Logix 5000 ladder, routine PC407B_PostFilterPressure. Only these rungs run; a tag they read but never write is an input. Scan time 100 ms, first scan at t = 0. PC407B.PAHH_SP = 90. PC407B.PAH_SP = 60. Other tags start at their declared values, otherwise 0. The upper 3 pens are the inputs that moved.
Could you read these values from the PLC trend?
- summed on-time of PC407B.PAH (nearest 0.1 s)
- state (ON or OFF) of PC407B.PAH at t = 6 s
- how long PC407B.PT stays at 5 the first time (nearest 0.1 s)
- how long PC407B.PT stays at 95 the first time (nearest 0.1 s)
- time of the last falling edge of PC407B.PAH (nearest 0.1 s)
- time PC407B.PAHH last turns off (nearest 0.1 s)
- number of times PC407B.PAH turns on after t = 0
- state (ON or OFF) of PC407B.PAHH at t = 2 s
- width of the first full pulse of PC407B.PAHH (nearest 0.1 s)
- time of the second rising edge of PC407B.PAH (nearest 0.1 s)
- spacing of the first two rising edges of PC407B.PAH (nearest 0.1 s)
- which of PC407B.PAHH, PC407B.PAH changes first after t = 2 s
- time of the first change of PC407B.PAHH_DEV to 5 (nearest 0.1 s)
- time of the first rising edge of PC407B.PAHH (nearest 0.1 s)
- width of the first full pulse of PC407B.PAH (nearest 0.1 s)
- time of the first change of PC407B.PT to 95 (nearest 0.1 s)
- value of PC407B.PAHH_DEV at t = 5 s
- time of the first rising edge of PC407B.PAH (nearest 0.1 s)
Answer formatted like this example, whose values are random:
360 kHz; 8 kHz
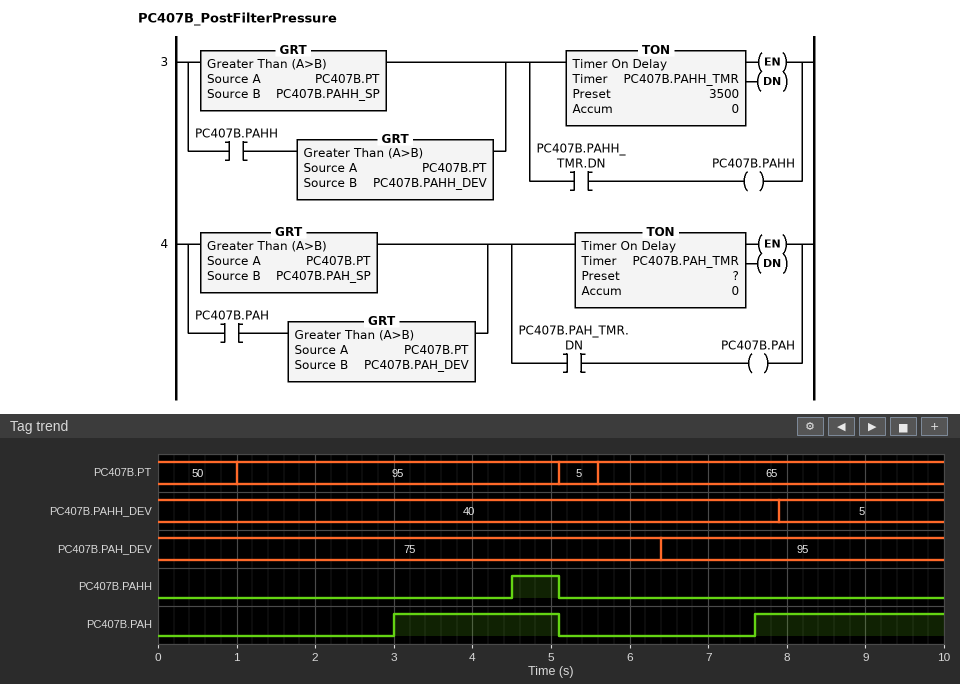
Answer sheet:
4.5 s; OFF; 0.5 s; 4.1 s; 5.1 s; 5.1 s; 2; OFF; 0.6 s; 7.6 s; 4.6 s; PC407B.PAH; 7.9 s; 4.5 s; 2.1 s; 1.0 s; 40; 3.0 s
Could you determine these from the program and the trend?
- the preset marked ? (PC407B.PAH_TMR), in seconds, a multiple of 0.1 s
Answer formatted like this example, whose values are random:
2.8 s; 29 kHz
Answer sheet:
2.0 s
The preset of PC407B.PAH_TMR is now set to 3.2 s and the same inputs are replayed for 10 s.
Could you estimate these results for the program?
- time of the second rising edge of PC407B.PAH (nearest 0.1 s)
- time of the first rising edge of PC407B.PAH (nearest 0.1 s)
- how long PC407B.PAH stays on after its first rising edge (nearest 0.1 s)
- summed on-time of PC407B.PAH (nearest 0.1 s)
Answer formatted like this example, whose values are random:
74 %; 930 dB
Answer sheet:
8.8 s; 4.2 s; 0.9 s; 2.1 s
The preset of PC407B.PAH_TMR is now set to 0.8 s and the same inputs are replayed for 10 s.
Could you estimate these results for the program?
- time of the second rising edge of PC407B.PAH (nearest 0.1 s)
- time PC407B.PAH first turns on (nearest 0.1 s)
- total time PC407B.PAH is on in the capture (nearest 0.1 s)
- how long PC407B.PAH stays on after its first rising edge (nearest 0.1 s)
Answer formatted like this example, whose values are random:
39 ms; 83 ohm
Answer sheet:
6.4 s; 1.8 s; 6.9 s; 3.3 s
